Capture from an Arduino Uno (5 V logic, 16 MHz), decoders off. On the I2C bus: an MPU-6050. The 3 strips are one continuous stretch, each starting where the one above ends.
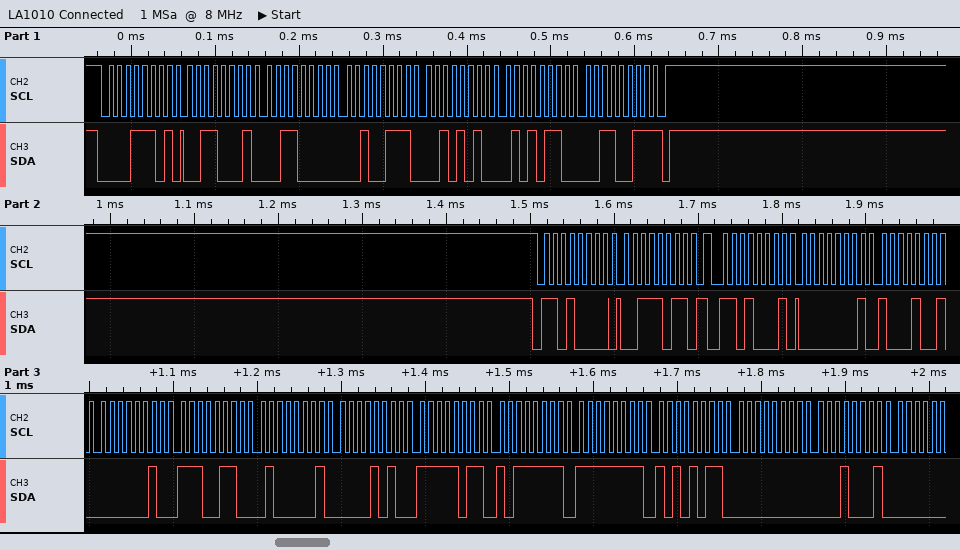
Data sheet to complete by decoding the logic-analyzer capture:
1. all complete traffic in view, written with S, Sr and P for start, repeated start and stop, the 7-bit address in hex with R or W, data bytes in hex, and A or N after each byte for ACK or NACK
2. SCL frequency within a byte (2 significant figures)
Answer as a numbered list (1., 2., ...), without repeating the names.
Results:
1. S 0ER A 31 A 30 A 27 A 2A A 56 A 33 N P S 68W A 3B A Sr 68R A 01 A 89 A 02 A E6 A 41 A 0A A FB A BF A FF A AB A 00 A 11 A
2. 100 kHz
